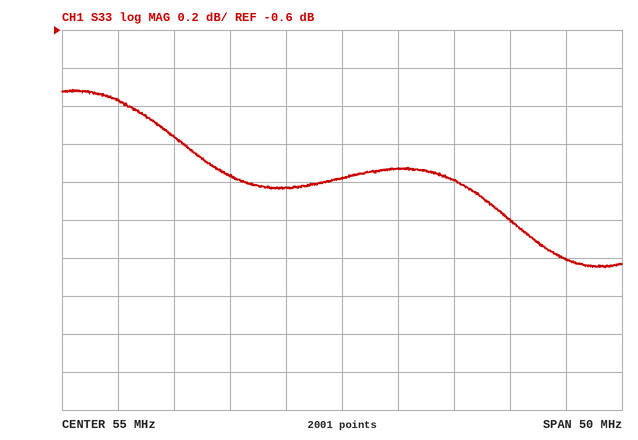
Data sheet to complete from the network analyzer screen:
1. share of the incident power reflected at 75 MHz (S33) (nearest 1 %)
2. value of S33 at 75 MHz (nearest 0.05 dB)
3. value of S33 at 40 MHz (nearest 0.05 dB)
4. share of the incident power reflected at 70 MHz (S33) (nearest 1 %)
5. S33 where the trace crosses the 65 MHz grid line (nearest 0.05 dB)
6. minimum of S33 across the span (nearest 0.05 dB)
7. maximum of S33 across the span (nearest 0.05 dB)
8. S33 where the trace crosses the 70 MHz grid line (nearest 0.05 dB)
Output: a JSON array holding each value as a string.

["66 %", "-1.80 dB", "-1.15 dB", "69 %", "-1.40 dB", "-1.85 dB", "-0.90 dB", "-1.60 dB"]
